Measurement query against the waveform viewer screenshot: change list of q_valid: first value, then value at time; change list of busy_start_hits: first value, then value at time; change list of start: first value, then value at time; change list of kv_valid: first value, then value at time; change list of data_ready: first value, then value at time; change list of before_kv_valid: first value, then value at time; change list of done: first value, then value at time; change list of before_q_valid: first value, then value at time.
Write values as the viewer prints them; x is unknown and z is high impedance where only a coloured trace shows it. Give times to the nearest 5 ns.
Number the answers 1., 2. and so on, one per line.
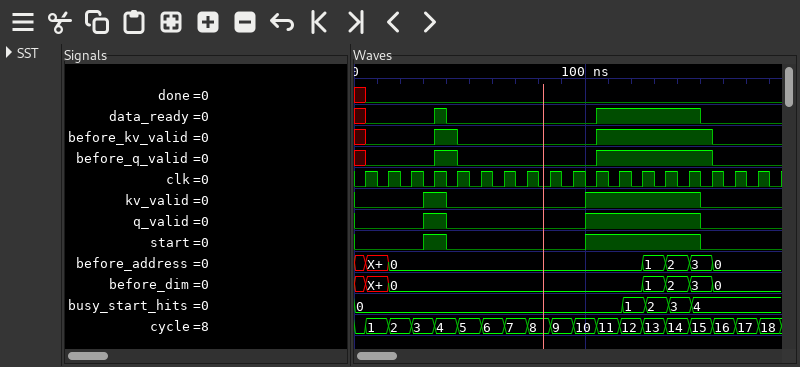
1. 0, 1 at 30 ns, 0 at 40 ns, 1 at 100 ns, 0 at 150 ns
2. 0, 1 at 115 ns, 2 at 125 ns, 3 at 135 ns, 4 at 145 ns
3. 0, 1 at 30 ns, 0 at 40 ns, 1 at 100 ns, 0 at 150 ns
4. 0, 1 at 30 ns, 0 at 40 ns, 1 at 100 ns, 0 at 150 ns
5. x, 0 at 5 ns, 1 at 35 ns, 0 at 40 ns, 1 at 105 ns, 0 at 150 ns
6. x, 0 at 5 ns, 1 at 35 ns, 0 at 45 ns, 1 at 105 ns, 0 at 155 ns
7. x, 0 at 5 ns
8. x, 0 at 5 ns, 1 at 35 ns, 0 at 45 ns, 1 at 105 ns, 0 at 155 ns
